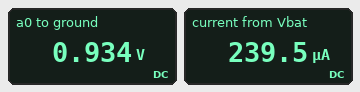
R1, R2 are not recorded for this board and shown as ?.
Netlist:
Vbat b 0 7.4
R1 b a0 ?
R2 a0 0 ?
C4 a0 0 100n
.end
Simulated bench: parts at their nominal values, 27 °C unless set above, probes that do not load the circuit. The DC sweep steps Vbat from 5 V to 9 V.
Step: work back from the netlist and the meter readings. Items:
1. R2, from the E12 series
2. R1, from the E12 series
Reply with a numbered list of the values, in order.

1. 3.9 kΩ
2. 27 kΩ
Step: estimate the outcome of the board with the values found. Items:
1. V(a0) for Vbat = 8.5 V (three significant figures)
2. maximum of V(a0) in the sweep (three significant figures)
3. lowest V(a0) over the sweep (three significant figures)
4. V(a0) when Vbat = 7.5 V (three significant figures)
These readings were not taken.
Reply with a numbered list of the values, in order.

1. 1.07 V
2. 1.14 V
3. 631 mV
4. 947 mV
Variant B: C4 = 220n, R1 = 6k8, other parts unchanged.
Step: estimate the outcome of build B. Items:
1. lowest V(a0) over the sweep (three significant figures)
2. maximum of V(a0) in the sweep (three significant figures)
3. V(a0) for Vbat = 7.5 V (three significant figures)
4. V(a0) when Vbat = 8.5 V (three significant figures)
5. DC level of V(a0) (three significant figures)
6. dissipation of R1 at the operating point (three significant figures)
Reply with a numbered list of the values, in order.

1. 1.82 V
2. 3.28 V
3. 2.73 V
4. 3.10 V
5. 2.70 V
6. 3.25 mW
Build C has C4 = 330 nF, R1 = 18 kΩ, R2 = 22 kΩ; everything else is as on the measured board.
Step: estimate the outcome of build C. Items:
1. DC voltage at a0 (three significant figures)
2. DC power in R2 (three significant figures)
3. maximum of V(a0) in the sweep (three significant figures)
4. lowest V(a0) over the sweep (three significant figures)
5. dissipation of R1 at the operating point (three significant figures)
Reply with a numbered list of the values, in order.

1. 4.07 V
2. 753 µW
3. 4.95 V
4. 2.75 V
5. 616 µW
